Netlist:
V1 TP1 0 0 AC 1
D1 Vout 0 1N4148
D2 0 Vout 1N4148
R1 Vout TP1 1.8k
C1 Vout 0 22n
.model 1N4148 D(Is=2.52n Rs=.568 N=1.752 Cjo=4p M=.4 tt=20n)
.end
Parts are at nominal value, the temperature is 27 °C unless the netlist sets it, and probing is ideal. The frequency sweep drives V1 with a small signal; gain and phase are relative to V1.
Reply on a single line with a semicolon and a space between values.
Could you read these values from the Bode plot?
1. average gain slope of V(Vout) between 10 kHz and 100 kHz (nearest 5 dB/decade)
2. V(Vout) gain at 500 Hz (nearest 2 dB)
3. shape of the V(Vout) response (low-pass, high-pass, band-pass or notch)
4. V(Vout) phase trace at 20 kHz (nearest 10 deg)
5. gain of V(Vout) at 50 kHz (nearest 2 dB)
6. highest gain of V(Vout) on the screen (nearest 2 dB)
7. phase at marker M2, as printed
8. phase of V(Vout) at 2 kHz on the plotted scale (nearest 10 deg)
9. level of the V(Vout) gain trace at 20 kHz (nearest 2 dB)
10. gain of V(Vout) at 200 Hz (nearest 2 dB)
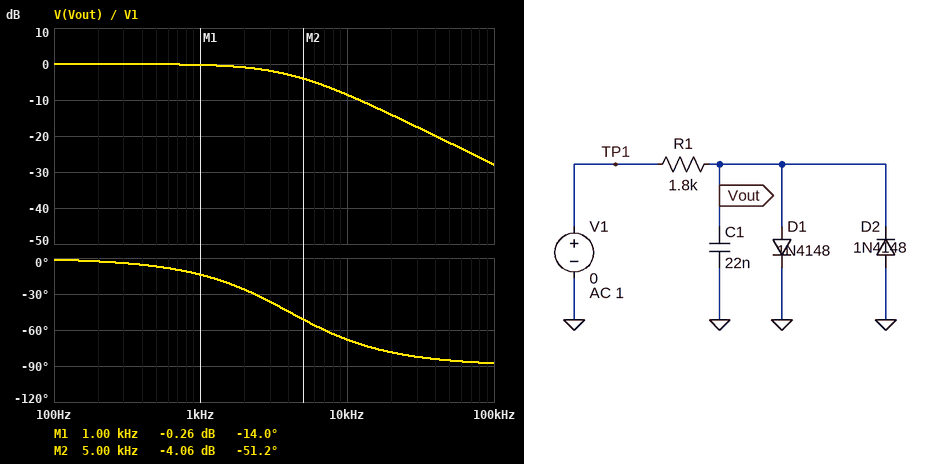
-20 dB/decade; 0 dB; low-pass; -80 deg; -22 dB; 0 dB; -51.2 deg; -30 deg; -14 dB; 0 dB
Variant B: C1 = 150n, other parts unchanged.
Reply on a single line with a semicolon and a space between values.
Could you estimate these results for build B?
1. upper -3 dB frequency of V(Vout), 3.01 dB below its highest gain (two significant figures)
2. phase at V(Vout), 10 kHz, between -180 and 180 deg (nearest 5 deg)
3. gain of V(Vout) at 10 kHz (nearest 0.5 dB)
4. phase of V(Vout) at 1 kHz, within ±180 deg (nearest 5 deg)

590 Hz; -85 deg; -24.5 dB; -60 deg
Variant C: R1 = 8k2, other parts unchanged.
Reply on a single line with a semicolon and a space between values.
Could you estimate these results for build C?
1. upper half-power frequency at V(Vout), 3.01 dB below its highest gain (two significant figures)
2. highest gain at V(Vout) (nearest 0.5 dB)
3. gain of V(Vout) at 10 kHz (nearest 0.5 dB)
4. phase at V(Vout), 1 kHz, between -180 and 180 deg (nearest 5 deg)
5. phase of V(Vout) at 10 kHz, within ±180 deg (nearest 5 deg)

880 Hz; 0 dB; -21.0 dB; -50 deg; -85 deg
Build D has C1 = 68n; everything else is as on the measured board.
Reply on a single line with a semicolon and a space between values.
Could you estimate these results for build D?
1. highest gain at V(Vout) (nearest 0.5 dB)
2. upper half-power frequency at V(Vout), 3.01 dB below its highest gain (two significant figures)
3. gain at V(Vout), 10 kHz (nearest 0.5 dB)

0 dB; 1.3 kHz; -18.0 dB
